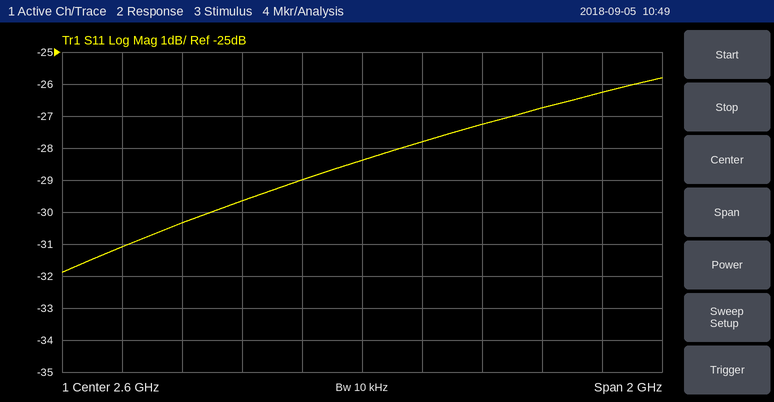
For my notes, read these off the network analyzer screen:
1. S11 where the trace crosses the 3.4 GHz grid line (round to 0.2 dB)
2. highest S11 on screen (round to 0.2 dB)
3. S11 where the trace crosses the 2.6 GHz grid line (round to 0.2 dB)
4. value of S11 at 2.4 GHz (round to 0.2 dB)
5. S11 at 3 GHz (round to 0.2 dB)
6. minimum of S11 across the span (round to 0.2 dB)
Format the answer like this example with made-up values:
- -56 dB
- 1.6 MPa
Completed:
- -26.2 dB
- -25.8 dB
- -28.4 dB
- -29.0 dB
- -27.2 dB
- -31.8 dB
